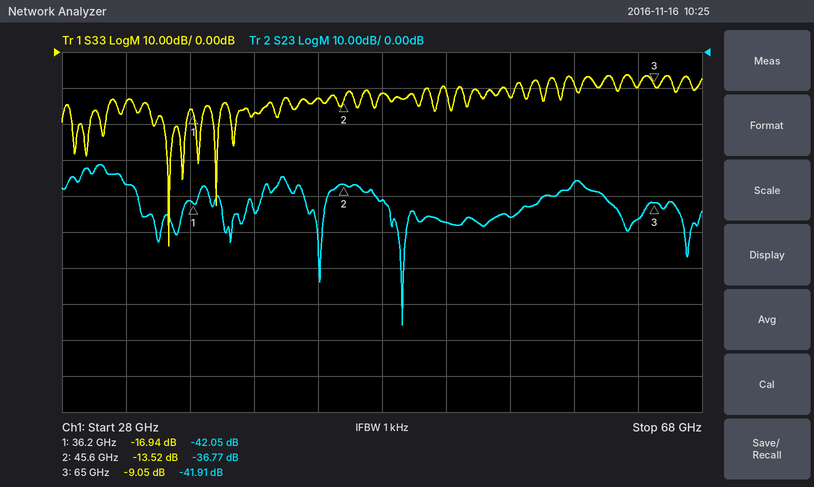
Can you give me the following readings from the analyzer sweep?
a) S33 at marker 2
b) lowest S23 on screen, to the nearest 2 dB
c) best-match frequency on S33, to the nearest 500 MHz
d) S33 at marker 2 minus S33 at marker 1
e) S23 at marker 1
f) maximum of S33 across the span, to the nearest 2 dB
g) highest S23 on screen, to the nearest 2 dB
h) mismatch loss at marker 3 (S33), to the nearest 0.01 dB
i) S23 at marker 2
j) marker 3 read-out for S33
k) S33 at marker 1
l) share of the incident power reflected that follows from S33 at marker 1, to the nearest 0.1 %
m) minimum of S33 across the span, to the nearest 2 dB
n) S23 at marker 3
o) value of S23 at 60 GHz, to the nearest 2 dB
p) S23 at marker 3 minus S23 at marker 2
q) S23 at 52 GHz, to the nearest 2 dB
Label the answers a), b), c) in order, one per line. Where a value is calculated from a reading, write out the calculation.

a) -13.52 dB
b) -76 dB
c) 34.5 GHz
d) -13.52 − (-16.94) = 3.42 dB
e) -42.05 dB
f) -6 dB
g) -32 dB
h) −10 log10(1 − 10^(-9.05/10)) ≈ 0.58 dB
i) -36.77 dB
j) -9.05 dB
k) -16.94 dB
l) 10^(-16.94/10) ≈ 2.0 %
m) -54 dB
n) -41.91 dB
o) -36 dB
p) -41.91 − (-36.77) = -5.14 dB
q) -48 dB
